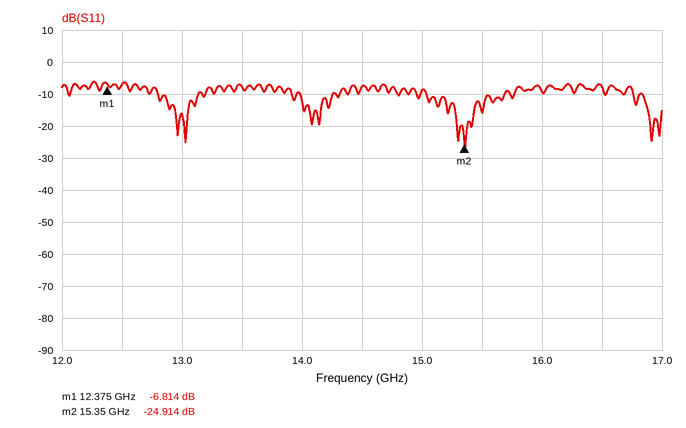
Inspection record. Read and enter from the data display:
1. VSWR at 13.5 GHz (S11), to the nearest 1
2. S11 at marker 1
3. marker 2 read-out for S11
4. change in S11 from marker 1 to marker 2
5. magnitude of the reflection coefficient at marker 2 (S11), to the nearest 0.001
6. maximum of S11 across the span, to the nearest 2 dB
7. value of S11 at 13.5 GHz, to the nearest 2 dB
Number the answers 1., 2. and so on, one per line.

1. 2
2. -6.814 dB
3. -24.914 dB
4. -18.100 dB
5. 0.057
6. -6 dB
7. -8 dB
